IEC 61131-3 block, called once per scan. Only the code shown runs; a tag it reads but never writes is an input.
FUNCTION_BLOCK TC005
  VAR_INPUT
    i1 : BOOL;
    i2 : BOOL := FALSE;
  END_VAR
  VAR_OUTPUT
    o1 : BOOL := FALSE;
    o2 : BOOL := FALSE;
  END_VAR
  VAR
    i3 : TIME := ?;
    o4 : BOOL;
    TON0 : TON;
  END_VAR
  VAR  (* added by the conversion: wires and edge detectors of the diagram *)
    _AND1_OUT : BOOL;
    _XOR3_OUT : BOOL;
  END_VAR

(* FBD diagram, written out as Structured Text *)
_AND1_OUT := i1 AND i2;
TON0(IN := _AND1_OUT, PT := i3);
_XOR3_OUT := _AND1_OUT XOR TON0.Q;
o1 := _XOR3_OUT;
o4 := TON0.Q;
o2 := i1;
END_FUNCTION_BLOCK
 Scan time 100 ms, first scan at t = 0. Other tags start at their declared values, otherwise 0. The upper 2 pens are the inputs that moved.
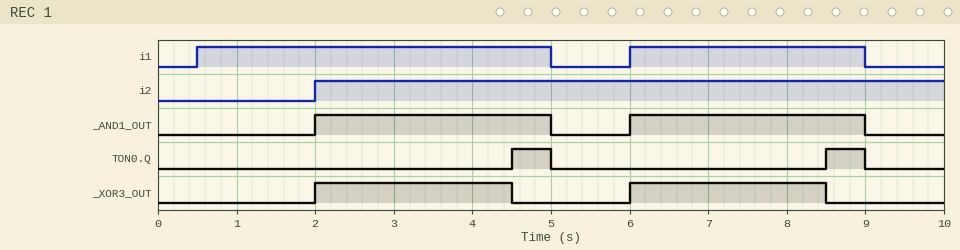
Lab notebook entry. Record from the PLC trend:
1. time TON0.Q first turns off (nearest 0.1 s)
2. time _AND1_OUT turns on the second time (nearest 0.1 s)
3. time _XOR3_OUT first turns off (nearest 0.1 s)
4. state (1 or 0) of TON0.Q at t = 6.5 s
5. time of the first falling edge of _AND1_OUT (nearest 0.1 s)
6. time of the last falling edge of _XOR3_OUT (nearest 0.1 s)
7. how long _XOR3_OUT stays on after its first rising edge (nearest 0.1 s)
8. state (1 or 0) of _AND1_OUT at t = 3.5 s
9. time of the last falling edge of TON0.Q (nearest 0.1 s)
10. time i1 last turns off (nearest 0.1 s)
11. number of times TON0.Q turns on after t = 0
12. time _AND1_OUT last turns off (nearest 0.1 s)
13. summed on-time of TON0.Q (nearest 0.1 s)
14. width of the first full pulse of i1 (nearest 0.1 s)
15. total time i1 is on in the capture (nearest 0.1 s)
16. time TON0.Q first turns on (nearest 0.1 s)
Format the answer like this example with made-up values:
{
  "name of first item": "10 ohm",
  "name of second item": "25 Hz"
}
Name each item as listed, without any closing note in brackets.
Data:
{
  "time TON0.Q first turns off": "5.0 s",
  "time _AND1_OUT turns on the second time": "6.0 s",
  "time _XOR3_OUT first turns off": "4.5 s",
  "state (1 or 0) of TON0.Q at t = 6.5 s": "0",
  "time of the first falling edge of _AND1_OUT": "5.0 s",
  "time of the last falling edge of _XOR3_OUT": "8.5 s",
  "how long _XOR3_OUT stays on after its first rising edge": "2.5 s",
  "state (1 or 0) of _AND1_OUT at t = 3.5 s": "1",
  "time of the last falling edge of TON0.Q": "9.0 s",
  "time i1 last turns off": "9.0 s",
  "number of times TON0.Q turns on after t = 0": "2",
  "time _AND1_OUT last turns off": "9.0 s",
  "summed on-time of TON0.Q": "1.0 s",
  "width of the first full pulse of i1": "4.5 s",
  "total time i1 is on in the capture": "7.5 s",
  "time TON0.Q first turns on": "4.5 s"
}
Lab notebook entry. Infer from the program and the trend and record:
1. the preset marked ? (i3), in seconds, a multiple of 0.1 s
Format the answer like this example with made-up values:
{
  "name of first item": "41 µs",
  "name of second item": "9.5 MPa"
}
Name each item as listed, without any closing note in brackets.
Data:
{
  "the preset marked ? (i3), in seconds, a multiple of 0.1 s": "2.5 s"
}
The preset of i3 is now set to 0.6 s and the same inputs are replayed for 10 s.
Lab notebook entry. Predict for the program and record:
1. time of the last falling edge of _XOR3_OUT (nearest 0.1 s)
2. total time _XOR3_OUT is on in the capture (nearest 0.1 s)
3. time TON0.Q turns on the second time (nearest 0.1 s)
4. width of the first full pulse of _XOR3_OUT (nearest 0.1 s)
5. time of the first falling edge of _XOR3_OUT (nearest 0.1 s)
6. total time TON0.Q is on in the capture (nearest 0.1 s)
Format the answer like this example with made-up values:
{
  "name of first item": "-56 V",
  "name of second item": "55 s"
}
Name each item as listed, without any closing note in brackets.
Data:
{
  "time of the last falling edge of _XOR3_OUT": "6.6 s",
  "total time _XOR3_OUT is on in the capture": "1.2 s",
  "time TON0.Q turns on the second time": "6.6 s",
  "width of the first full pulse of _XOR3_OUT": "0.6 s",
  "time of the first falling edge of _XOR3_OUT": "2.6 s",
  "total time TON0.Q is on in the capture": "4.8 s"
}
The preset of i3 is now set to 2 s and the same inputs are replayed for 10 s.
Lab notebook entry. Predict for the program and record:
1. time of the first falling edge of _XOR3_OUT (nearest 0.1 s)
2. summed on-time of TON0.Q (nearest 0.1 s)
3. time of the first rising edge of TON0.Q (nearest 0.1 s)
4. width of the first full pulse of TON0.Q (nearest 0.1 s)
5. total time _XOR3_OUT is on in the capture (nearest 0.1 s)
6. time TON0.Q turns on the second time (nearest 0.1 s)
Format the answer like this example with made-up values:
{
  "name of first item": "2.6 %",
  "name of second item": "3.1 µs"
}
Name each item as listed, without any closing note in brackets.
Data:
{
  "time of the first falling edge of _XOR3_OUT": "4.0 s",
  "summed on-time of TON0.Q": "2.0 s",
  "time of the first rising edge of TON0.Q": "4.0 s",
  "width of the first full pulse of TON0.Q": "1.0 s",
  "total time _XOR3_OUT is on in the capture": "4.0 s",
  "time TON0.Q turns on the second time": "8.0 s"
}
